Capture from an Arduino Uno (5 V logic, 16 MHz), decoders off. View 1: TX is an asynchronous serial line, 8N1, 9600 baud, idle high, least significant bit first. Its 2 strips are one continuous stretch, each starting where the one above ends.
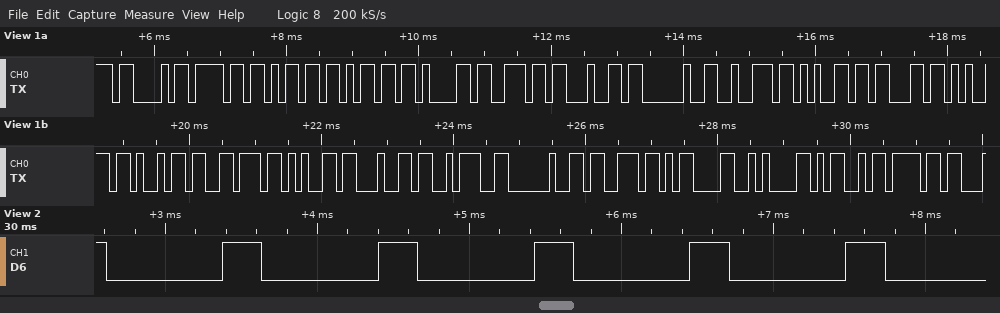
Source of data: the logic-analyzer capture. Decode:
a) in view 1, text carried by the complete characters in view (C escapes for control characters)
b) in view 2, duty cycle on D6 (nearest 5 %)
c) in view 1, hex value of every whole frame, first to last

"Command received: s\r\nMo"
25 %
43 6F 6D 6D 61 6E 64 20 72 65 63 65 69 76 65 64 3A 20 73 0D 0A 4D 6F
